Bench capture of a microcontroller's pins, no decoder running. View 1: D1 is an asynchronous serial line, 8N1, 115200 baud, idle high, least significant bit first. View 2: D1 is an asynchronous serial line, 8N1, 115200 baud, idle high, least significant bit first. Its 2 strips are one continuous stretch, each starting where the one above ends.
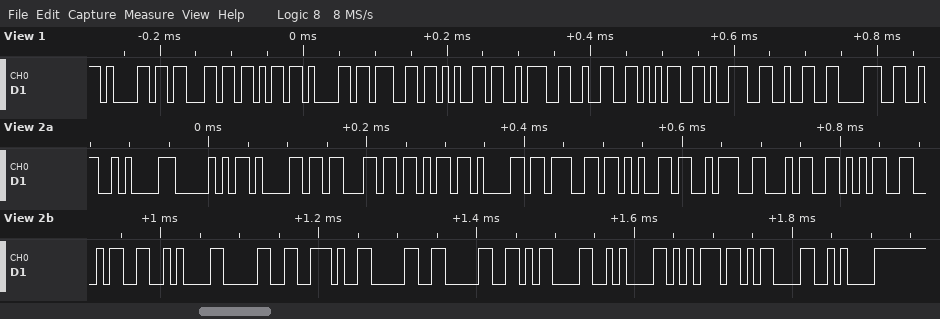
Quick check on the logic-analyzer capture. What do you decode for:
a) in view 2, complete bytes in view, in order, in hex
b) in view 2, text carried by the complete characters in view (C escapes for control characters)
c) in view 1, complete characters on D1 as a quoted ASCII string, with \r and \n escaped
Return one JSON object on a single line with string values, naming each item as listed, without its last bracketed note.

{"in view 2, complete bytes in view, in order, in hex": "0A 50 61 63 6B 61 67 65 3A 34 35 34 0A 30 2E 30 30 0D 0A 75 0D 0A", "in view 2, text carried by the complete characters in view": "\"\\nPackage:454\\n0.00\\r\\nu\\r\\n\"", "in view 1, complete characters on D1 as a quoted ASCII string, with \\r and \\n escaped": "\"ackage:25928\""}
